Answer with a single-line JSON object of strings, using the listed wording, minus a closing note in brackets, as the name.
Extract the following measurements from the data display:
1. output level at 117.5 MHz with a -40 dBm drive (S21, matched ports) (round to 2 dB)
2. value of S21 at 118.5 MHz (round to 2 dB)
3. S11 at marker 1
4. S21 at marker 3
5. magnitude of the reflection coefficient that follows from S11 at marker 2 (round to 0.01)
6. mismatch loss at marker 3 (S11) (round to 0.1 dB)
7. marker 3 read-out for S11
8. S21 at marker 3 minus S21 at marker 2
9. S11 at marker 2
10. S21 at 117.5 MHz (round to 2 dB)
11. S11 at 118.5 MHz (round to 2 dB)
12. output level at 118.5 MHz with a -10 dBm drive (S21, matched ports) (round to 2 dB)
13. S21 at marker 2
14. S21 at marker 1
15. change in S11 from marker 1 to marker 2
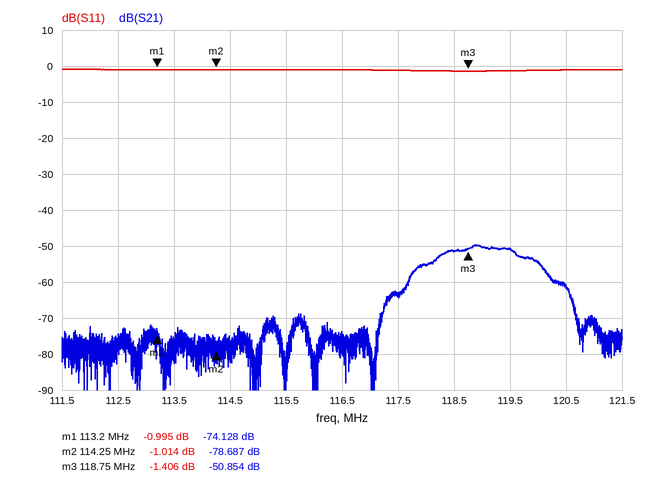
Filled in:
{"output level at 117.5 MHz with a -40 dBm drive (S21, matched ports)": "-104 dBm", "value of S21 at 118.5 MHz": "-52 dB", "S11 at marker 1": "-0.995 dB", "S21 at marker 3": "-50.854 dB", "magnitude of the reflection coefficient that follows from S11 at marker 2": "0.89", "mismatch loss at marker 3 (S11)": "5.6 dB", "marker 3 read-out for S11": "-1.406 dB", "S21 at marker 3 minus S21 at marker 2": "27.833 dB", "S11 at marker 2": "-1.014 dB", "S21 at 117.5 MHz": "-64 dB", "S11 at 118.5 MHz": "-2 dB", "output level at 118.5 MHz with a -10 dBm drive (S21, matched ports)": "-62 dBm", "S21 at marker 2": "-78.687 dB", "S21 at marker 1": "-74.128 dB", "change in S11 from marker 1 to marker 2": "-0.019 dB"}
